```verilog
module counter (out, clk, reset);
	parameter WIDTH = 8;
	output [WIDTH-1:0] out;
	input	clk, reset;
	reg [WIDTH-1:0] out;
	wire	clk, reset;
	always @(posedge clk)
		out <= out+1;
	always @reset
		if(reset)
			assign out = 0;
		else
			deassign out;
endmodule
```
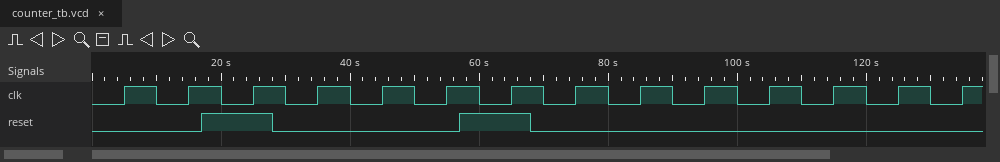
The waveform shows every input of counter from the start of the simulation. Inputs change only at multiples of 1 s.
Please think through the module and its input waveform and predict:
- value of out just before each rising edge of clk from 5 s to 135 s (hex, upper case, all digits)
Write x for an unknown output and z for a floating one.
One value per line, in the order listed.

x, x, 00, 00, 01, 02, 00, 00, 01, 02, 03, 04, 05, 06
